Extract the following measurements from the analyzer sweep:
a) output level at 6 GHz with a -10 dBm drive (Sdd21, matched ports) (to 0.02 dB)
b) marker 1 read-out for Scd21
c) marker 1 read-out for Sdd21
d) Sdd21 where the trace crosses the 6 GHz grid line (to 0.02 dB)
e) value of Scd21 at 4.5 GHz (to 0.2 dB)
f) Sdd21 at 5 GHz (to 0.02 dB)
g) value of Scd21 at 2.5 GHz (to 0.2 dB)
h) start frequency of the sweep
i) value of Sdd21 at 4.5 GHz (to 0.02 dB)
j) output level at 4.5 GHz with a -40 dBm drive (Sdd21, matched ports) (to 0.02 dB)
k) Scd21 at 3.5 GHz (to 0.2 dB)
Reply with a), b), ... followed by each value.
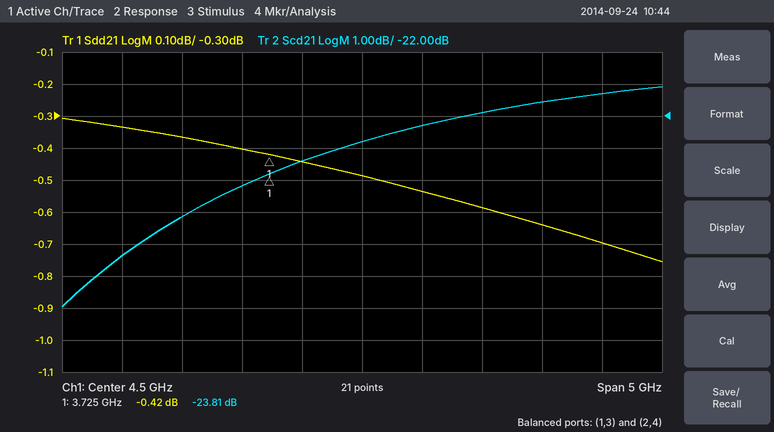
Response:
a) -10.64 dBm
b) -23.81 dB
c) -0.42 dB
d) -0.64 dB
e) -22.8 dB
f) -0.54 dB
g) -26.4 dB
h) 2 GHz
i) -0.48 dB
j) -40.48 dBm
k) -24.2 dB
